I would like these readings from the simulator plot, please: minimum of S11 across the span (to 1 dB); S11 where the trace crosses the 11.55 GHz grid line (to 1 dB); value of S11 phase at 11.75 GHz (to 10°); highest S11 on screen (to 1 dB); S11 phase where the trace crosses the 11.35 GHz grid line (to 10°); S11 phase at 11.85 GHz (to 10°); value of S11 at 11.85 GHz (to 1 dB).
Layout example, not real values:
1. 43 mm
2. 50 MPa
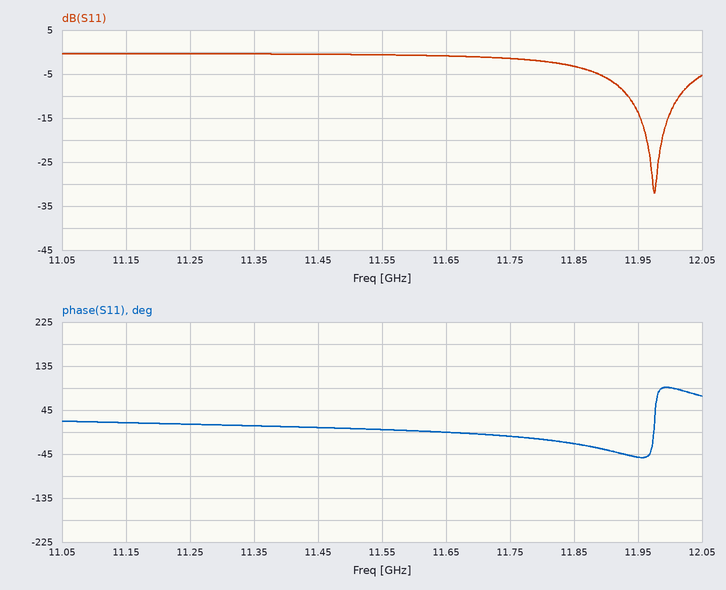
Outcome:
1. -32 dB
2. -1 dB
3. -10°
4. 0 dB
5. 10°
6. -20°
7. -3 dB
